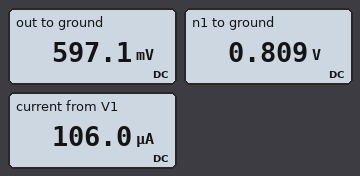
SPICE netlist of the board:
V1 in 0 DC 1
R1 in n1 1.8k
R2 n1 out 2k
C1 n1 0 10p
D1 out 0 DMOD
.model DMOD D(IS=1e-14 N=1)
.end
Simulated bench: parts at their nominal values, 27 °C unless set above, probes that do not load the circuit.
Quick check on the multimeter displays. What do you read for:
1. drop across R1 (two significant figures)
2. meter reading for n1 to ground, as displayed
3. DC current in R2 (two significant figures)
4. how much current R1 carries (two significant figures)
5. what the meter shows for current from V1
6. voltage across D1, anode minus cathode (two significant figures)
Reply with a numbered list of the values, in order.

1. 190 mV
2. 0.809 V
3. 110 µA
4. 110 µA
5. 106.0 µA
6. 600 mV
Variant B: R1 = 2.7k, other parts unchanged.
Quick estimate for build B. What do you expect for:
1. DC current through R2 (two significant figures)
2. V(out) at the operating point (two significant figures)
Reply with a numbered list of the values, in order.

1. 87 µA
2. 590 mV
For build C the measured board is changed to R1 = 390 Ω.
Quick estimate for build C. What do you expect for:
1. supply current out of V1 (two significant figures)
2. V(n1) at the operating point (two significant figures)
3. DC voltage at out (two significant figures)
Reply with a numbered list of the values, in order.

1. 160 µA
2. 940 mV
3. 610 mV
